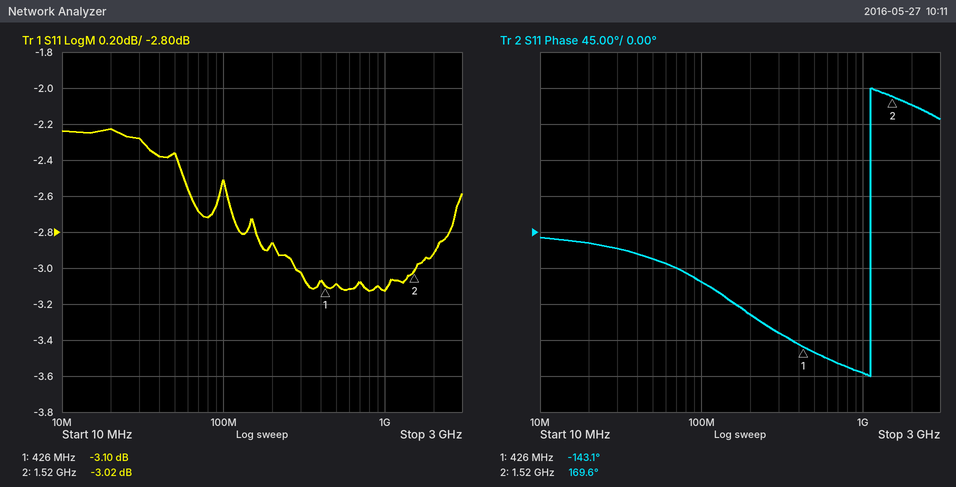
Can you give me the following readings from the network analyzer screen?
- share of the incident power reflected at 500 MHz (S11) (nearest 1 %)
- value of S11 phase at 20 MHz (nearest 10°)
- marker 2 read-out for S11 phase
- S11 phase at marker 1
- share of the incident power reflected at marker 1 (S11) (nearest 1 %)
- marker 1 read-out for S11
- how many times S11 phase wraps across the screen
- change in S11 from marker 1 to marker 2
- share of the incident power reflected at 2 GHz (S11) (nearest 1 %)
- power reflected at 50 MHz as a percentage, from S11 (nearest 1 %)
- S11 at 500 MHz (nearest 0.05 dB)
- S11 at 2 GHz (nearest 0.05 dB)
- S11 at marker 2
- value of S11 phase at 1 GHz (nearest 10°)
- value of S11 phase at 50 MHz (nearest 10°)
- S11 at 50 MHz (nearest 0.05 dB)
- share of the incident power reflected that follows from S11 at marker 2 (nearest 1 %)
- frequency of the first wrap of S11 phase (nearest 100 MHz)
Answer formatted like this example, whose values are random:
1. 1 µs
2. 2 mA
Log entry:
1. 49 %
2. -10°
3. 169.6°
4. -143.1°
5. 49 %
6. -3.10 dB
7. 1
8. 0.08 dB
9. 51 %
10. 58 %
11. -3.10 dB
12. -2.90 dB
13. -3.02 dB
14. -180°
15. -30°
16. -2.35 dB
17. 50 %
18. 1.1 GHz
